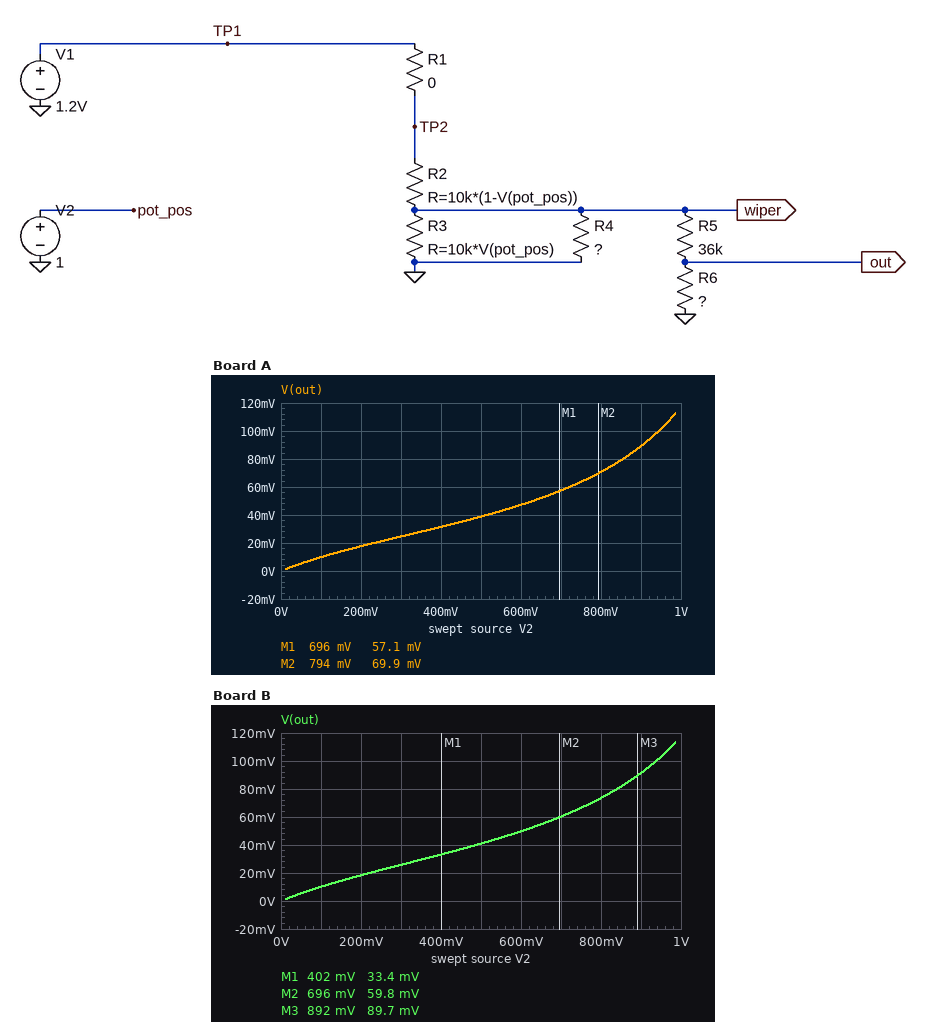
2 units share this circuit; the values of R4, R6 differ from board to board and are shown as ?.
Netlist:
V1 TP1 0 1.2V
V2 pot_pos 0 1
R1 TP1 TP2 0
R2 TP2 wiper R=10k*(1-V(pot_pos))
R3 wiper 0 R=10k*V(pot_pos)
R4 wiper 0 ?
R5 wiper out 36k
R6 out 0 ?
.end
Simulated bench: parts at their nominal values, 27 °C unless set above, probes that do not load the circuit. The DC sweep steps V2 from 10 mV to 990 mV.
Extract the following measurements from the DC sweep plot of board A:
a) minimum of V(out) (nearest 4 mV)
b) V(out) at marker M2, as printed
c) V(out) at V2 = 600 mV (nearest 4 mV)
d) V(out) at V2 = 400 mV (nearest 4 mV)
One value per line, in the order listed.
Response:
0 V
69.9 mV
48 mV
32 mV
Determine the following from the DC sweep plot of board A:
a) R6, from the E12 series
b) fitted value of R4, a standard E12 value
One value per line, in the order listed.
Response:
3.9 kΩ
5.6 kΩ
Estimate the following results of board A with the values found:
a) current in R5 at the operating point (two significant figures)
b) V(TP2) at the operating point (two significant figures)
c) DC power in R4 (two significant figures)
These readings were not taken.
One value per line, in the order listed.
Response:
30 µA
1.2 V
260 µW
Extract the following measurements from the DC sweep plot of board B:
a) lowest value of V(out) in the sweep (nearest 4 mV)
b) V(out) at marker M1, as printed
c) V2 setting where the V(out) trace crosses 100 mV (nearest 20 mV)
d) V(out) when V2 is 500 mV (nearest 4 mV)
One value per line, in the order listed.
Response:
0 V
33.4 mV
940 mV
40 mV
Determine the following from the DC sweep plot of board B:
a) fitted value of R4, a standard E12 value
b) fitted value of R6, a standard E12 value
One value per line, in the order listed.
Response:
6.8 kΩ
3.9 kΩ
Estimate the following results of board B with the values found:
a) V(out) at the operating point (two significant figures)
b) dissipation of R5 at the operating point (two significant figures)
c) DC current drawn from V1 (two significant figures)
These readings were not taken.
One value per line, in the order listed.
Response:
120 mV
33 µW
240 µA
